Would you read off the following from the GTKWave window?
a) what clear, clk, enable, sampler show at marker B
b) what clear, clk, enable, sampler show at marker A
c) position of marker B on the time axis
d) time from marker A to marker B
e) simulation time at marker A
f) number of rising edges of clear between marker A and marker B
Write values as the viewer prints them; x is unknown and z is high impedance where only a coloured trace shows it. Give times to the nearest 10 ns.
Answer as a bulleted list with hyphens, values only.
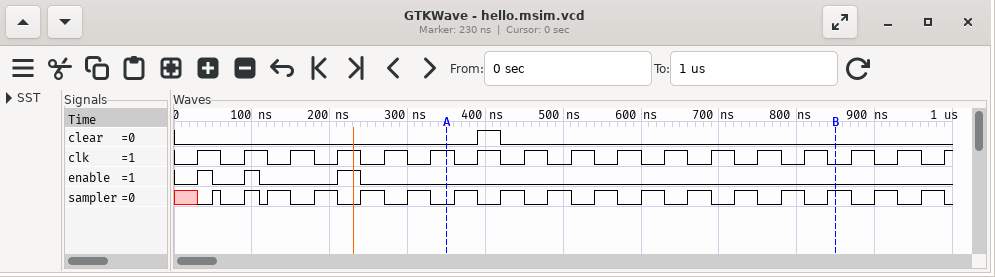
- clear=0, clk=0, enable=0, sampler=1
- clear=0, clk=1, enable=0, sampler=0
- 850 ns
- 500 ns
- 350 ns
- 1
